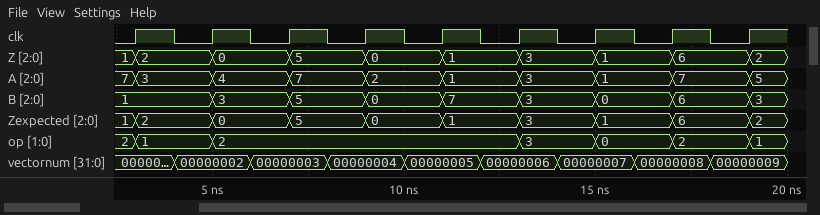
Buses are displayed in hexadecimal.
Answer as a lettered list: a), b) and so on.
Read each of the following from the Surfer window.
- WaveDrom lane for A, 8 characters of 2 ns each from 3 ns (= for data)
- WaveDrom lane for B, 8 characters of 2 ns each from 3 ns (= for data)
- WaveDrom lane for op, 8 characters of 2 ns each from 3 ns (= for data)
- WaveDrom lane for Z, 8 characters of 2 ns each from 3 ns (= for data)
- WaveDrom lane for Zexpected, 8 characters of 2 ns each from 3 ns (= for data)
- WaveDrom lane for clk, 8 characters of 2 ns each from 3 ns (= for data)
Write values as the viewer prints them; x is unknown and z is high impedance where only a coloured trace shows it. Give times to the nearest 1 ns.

a) {name: 'A', wave: '========', data: '3 4 7 2 1 3 1 7'}
b) {name: 'B', wave: '========', data: '1 3 5 0 7 3 0 6'}
c) {name: 'op', wave: '==...===', data: '1 2 3 0 2'}
d) {name: 'Z', wave: '========', data: '2 0 5 0 1 3 1 6'}
e) {name: 'Zexpected', wave: '========', data: '2 0 5 0 1 3 1 6'}
f) {name: 'clk', wave: 'p.......'}
